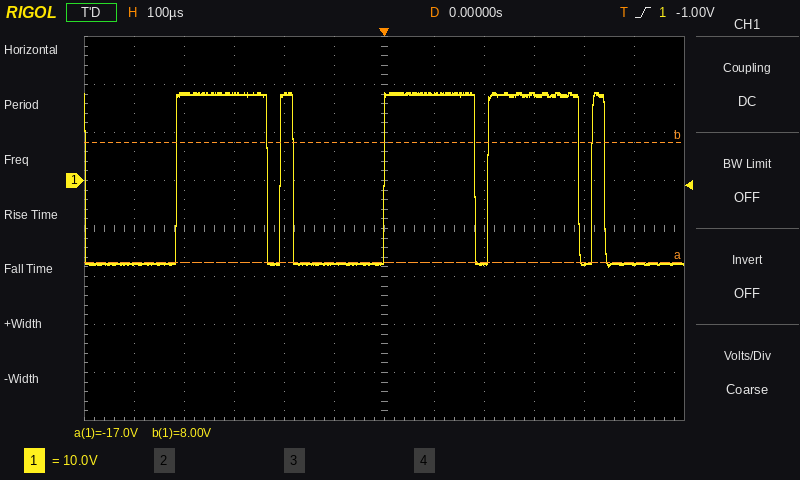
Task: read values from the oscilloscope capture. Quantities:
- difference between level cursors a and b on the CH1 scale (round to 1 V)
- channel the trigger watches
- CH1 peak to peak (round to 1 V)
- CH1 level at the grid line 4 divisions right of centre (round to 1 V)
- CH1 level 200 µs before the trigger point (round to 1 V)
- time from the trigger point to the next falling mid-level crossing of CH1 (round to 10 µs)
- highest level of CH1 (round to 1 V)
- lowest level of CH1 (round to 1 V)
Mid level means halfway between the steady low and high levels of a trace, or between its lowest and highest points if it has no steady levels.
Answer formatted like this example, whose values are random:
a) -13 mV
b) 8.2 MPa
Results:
a) 25 V
b) CH1
c) 36 V
d) -17 V
e) 18 V
f) 180 µs
g) 18 V
h) -18 V
